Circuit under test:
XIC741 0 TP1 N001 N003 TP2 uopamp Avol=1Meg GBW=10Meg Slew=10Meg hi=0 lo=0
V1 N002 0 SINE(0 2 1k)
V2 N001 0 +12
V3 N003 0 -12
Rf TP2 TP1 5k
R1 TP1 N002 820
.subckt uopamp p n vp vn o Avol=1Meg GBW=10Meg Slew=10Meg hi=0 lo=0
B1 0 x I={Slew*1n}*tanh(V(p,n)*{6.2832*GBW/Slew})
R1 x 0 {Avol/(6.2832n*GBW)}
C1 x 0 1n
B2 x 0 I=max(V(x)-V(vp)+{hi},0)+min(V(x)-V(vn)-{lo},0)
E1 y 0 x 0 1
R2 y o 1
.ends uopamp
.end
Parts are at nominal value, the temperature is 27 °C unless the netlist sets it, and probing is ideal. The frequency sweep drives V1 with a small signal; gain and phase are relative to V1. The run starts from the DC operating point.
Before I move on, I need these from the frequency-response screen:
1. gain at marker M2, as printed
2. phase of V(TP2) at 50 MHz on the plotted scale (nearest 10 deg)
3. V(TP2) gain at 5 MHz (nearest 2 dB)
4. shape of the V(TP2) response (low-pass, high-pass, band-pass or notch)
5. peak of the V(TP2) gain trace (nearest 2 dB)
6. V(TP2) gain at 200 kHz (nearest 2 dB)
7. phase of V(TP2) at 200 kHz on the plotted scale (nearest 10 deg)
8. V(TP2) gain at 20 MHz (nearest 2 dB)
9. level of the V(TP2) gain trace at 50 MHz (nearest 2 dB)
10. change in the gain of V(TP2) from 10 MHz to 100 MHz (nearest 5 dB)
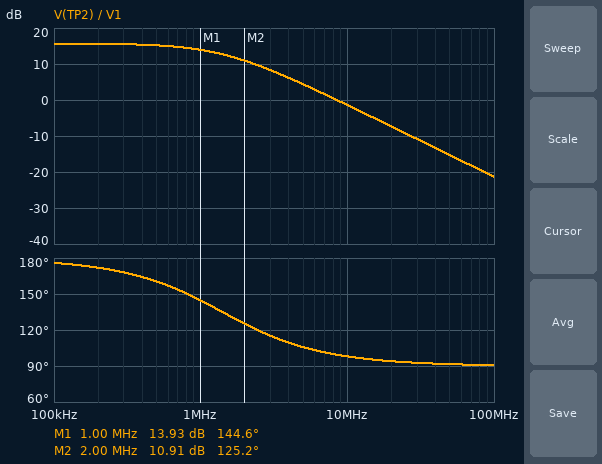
10.91 dB
90 deg
4 dB
low-pass
16 dB
16 dB
170 deg
-8 dB
-16 dB
-20 dB
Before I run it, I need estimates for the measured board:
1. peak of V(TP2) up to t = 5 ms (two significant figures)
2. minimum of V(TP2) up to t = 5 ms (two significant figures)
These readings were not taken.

12 V
-12 V
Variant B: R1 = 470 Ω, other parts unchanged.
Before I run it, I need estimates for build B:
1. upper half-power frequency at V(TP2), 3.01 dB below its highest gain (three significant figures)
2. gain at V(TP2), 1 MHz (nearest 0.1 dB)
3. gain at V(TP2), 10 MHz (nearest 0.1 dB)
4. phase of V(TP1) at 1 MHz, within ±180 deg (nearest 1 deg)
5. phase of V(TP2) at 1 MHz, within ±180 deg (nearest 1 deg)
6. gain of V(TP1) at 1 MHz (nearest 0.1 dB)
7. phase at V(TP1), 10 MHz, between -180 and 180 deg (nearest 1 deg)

859 kHz
16.8 dB
-0.8 dB
41 deg
131 deg
-3.2 dB
5 deg
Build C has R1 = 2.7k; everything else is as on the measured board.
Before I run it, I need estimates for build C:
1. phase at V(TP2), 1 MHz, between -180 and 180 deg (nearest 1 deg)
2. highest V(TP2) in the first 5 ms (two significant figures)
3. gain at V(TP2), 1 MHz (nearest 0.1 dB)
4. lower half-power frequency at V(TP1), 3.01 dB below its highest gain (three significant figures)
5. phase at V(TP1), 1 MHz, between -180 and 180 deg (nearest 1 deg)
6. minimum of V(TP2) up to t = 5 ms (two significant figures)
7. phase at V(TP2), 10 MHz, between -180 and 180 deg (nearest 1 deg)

164 deg
3.7 V
5.0 dB
3.51 MHz
74 deg
-3.7 V
109 deg
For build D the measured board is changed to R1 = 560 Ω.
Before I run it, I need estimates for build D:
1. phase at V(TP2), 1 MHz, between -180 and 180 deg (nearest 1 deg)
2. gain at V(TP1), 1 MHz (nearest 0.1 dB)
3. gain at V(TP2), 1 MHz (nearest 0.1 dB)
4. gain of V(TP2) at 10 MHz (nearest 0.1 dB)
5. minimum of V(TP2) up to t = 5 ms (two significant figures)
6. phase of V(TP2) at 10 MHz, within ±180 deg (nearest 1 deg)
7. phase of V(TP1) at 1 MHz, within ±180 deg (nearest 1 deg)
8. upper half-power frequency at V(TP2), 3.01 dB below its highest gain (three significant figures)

135 deg
-4.0 dB
16.0 dB
-1.0 dB
-12 V
96 deg
45 deg
1.01 MHz
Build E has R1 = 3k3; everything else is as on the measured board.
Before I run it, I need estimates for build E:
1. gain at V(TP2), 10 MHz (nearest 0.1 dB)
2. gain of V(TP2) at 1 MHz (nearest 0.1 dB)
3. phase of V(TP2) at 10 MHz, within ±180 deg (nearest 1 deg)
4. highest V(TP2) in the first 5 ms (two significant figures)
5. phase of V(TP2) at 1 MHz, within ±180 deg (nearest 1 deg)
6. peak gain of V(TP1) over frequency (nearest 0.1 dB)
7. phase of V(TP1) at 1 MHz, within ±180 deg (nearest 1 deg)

-5.0 dB
3.3 dB
112 deg
3.0 V
166 deg
-4.4 dB
76 deg
